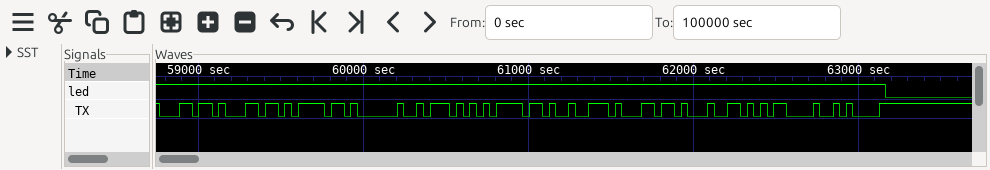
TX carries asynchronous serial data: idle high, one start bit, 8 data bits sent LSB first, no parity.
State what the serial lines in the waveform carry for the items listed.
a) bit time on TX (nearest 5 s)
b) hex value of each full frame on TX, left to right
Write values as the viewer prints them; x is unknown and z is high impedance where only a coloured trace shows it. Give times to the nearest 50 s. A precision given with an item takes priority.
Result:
40 s
6C, 6C, 6F, 20, 57, 6F, 72, 6C, 64, 0D, 0A
